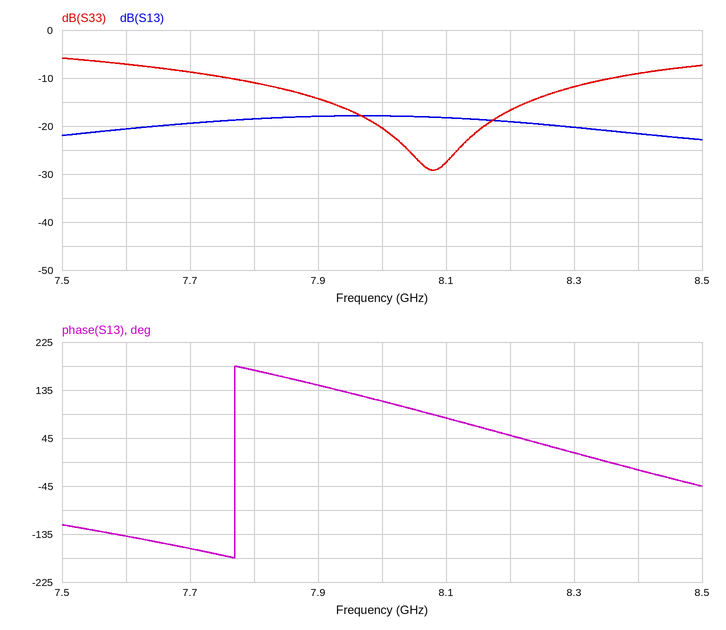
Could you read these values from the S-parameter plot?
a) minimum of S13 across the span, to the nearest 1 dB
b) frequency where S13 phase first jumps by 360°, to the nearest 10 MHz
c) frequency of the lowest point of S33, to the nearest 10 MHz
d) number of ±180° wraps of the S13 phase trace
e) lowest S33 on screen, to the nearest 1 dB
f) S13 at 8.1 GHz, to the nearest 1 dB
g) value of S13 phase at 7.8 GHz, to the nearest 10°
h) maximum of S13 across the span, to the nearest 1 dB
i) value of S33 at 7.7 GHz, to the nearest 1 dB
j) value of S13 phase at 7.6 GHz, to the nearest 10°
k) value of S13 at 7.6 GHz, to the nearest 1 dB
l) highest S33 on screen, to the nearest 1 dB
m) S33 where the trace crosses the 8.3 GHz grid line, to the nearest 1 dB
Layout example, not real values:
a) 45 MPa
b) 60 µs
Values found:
a) -23 dB
b) 7.77 GHz
c) 8.08 GHz
d) 1
e) -29 dB
f) -18 dB
g) 170°
h) -18 dB
i) -9 dB
j) -140°
k) -21 dB
l) -6 dB
m) -12 dB
